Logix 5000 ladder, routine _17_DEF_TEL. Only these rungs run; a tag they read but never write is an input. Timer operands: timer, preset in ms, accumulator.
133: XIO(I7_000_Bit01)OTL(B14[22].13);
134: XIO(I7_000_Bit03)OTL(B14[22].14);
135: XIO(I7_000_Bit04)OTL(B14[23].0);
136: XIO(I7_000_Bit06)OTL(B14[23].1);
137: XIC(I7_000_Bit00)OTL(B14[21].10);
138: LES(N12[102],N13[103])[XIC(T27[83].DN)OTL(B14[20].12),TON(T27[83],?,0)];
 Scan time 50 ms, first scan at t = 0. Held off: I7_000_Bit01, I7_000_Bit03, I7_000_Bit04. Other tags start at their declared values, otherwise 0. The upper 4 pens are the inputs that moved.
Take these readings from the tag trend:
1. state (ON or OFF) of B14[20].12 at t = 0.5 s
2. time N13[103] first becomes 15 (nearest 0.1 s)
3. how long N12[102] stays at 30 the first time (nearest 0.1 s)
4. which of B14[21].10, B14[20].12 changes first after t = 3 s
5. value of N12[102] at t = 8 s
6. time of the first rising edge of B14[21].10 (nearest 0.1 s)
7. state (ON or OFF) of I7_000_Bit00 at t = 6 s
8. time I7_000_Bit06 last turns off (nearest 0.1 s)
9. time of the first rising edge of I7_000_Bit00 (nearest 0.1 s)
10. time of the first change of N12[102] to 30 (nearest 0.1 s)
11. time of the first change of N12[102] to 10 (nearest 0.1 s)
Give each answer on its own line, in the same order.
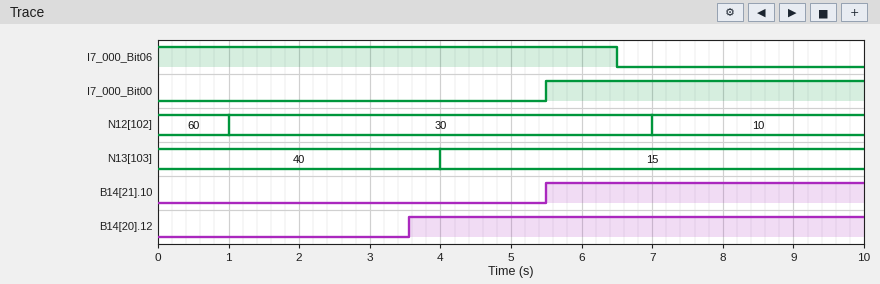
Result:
OFF
4.0 s
6.0 s
B14[20].12
10
5.5 s
ON
6.5 s
5.5 s
1.0 s
7.0 s
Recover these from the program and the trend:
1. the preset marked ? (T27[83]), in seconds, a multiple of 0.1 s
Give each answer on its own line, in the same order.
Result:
2.5 s
